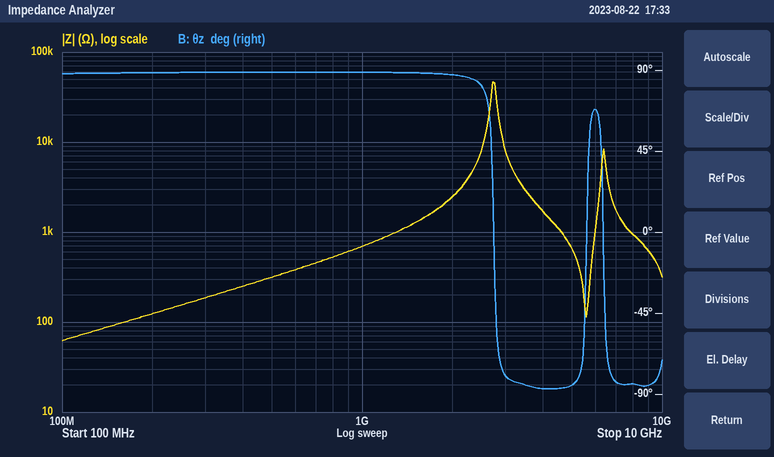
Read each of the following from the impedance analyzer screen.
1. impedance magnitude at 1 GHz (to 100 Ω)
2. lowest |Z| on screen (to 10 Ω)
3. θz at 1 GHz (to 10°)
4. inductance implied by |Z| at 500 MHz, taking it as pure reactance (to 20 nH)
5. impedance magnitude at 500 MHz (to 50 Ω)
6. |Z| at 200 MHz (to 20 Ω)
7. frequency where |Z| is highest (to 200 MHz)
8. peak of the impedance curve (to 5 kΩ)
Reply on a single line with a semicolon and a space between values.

700 Ω; 60 Ω; 90°; 100 nH; 300 Ω; 120 Ω; 2.8 GHz; 45 kΩ
